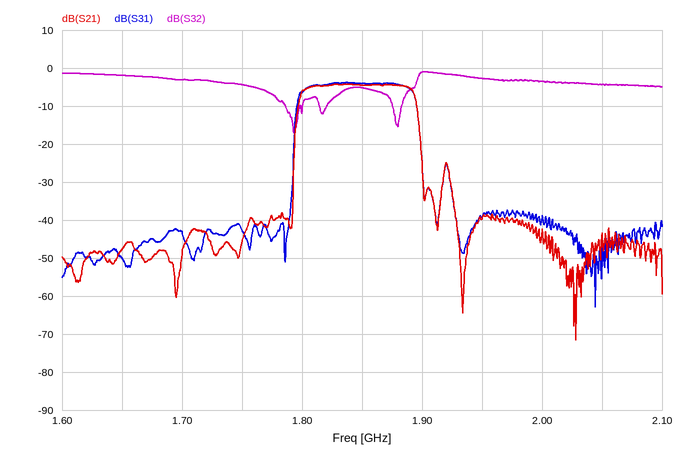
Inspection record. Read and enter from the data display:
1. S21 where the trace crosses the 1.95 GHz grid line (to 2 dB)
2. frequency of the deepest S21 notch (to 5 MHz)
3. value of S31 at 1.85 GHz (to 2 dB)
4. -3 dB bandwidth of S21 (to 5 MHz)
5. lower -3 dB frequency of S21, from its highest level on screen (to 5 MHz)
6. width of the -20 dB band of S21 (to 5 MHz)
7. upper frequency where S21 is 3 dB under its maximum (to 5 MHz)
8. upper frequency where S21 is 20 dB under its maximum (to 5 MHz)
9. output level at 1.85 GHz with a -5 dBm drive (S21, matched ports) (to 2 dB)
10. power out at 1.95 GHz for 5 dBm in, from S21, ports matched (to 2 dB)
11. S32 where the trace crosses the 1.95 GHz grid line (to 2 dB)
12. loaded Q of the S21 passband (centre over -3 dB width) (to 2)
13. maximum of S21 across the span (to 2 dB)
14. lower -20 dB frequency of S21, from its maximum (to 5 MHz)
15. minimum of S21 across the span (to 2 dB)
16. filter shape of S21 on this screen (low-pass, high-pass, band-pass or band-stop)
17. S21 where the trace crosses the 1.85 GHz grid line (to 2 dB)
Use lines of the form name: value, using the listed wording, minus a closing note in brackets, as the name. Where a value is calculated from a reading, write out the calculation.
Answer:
S21 where the trace crosses the 1.95 GHz grid line: -40 dB
frequency of the deepest S21 notch: 2.030 GHz
value of S31 at 1.85 GHz: -4 dB
-3 dB bandwidth of S21: 1.895 GHz − 1.800 GHz = 95 MHz
lower -3 dB frequency of S21, from its highest level on screen: 1.800 GHz
width of the -20 dB band of S21: 1.900 GHz − 1.795 GHz = 105 MHz
upper frequency where S21 is 3 dB under its maximum: 1.895 GHz
upper frequency where S21 is 20 dB under its maximum: 1.900 GHz
output level at 1.85 GHz with a -5 dBm drive (S21, matched ports): -5 dBm + (-4 dB) = -10 dBm
power out at 1.95 GHz for 5 dBm in, from S21, ports matched: 5 dBm + (-40 dB) = -34 dBm
S32 where the trace crosses the 1.95 GHz grid line: -2 dB
loaded Q of the S21 passband (centre over -3 dB width): 1.8475 GHz / 95 MHz ≈ 19.4, so 20 to the nearest 2
maximum of S21 across the span: -4 dB
lower -20 dB frequency of S21, from its maximum: 1.795 GHz
minimum of S21 across the span: -72 dB
filter shape of S21 on this screen: band-pass
S21 where the trace crosses the 1.85 GHz grid line: -4 dB
